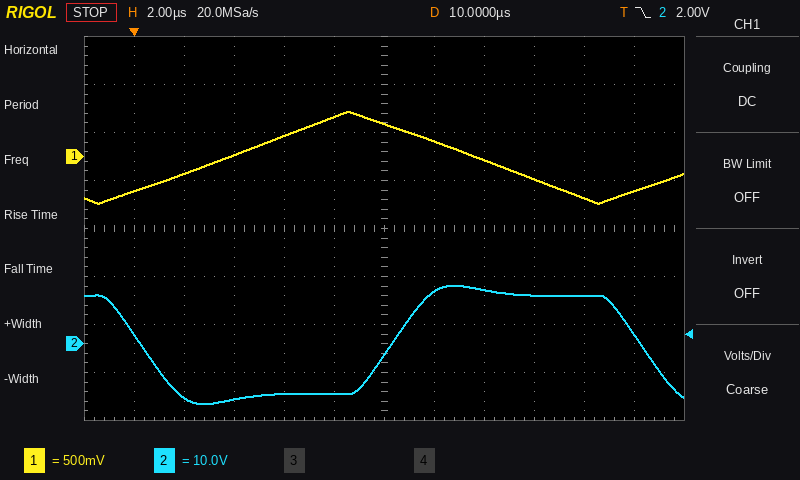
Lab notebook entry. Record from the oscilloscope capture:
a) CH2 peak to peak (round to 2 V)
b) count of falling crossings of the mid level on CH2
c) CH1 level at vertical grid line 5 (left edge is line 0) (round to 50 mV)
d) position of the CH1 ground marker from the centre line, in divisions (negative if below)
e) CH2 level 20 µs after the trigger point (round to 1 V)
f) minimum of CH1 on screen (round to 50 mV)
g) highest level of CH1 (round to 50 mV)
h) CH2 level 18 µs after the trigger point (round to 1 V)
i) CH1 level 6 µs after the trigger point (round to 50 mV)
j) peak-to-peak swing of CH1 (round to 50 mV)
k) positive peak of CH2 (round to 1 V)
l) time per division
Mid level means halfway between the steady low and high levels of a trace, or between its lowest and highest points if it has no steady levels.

24 V
2
400 mV
+1.5 div
2 V
-500 mV
450 mV
10 V
200 mV
950 mV
12 V
2 µs
